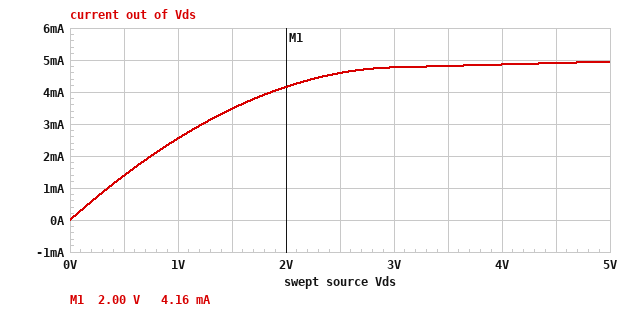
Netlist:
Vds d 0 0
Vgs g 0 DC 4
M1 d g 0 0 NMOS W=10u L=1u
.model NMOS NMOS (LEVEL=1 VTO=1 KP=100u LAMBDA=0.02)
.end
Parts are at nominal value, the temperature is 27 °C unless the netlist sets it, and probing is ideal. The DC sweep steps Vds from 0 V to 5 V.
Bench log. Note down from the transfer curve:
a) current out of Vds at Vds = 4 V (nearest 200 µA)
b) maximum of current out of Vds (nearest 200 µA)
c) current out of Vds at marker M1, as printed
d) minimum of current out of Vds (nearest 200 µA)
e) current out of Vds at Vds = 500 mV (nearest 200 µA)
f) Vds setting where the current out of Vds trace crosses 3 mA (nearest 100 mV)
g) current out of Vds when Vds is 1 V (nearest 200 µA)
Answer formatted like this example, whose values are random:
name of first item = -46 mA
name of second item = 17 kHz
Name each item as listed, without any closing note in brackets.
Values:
current out of Vds at Vds = 4 V = 4.8 mA
maximum of current out of Vds = 5.0 mA
current out of Vds at marker M1, as printed = 4.16 mA
minimum of current out of Vds = 0 A
current out of Vds at Vds = 500 mV = 1.4 mA
Vds setting where the current out of Vds trace crosses 3 mA = 1.2 V
current out of Vds when Vds is 1 V = 2.6 mA
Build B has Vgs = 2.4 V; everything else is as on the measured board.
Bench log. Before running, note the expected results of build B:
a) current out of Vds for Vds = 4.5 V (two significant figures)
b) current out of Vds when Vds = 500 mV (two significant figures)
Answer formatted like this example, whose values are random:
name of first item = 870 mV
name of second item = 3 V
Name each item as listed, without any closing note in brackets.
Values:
current out of Vds for Vds = 4.5 V = 1.1 mA
current out of Vds when Vds = 500 mV = 580 µA
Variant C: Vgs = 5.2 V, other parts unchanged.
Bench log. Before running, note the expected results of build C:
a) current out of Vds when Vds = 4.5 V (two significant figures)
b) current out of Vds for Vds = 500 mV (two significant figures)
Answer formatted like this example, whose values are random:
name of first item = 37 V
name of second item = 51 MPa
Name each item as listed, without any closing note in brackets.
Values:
current out of Vds when Vds = 4.5 V = 9.6 mA
current out of Vds for Vds = 500 mV = 2.0 mA
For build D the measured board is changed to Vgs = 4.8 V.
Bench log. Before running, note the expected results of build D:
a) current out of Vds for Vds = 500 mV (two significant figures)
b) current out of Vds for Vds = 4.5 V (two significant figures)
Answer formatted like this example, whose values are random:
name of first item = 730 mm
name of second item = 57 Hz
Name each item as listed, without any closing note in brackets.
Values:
current out of Vds for Vds = 500 mV = 1.8 mA
current out of Vds for Vds = 4.5 V = 7.9 mA
